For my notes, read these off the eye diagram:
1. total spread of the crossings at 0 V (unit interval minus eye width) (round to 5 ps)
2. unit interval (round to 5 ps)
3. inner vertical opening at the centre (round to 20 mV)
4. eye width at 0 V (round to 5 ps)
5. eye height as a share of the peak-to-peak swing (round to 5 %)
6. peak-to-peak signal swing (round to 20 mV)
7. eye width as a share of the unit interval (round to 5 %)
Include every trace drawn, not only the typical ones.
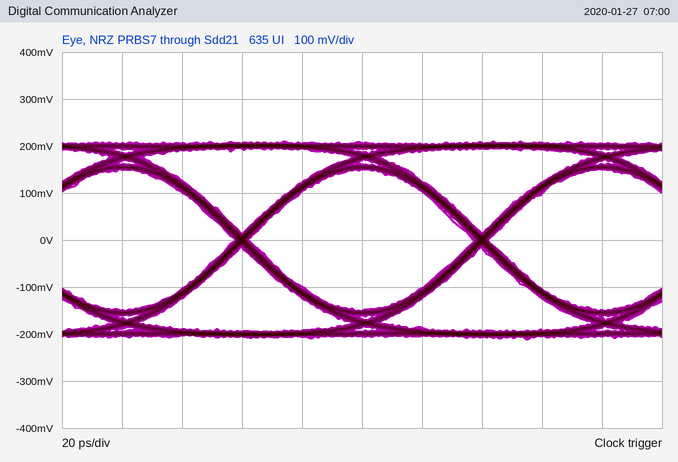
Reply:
5 ps
80 ps
300 mV
75 ps
70 %
420 mV
95 %
